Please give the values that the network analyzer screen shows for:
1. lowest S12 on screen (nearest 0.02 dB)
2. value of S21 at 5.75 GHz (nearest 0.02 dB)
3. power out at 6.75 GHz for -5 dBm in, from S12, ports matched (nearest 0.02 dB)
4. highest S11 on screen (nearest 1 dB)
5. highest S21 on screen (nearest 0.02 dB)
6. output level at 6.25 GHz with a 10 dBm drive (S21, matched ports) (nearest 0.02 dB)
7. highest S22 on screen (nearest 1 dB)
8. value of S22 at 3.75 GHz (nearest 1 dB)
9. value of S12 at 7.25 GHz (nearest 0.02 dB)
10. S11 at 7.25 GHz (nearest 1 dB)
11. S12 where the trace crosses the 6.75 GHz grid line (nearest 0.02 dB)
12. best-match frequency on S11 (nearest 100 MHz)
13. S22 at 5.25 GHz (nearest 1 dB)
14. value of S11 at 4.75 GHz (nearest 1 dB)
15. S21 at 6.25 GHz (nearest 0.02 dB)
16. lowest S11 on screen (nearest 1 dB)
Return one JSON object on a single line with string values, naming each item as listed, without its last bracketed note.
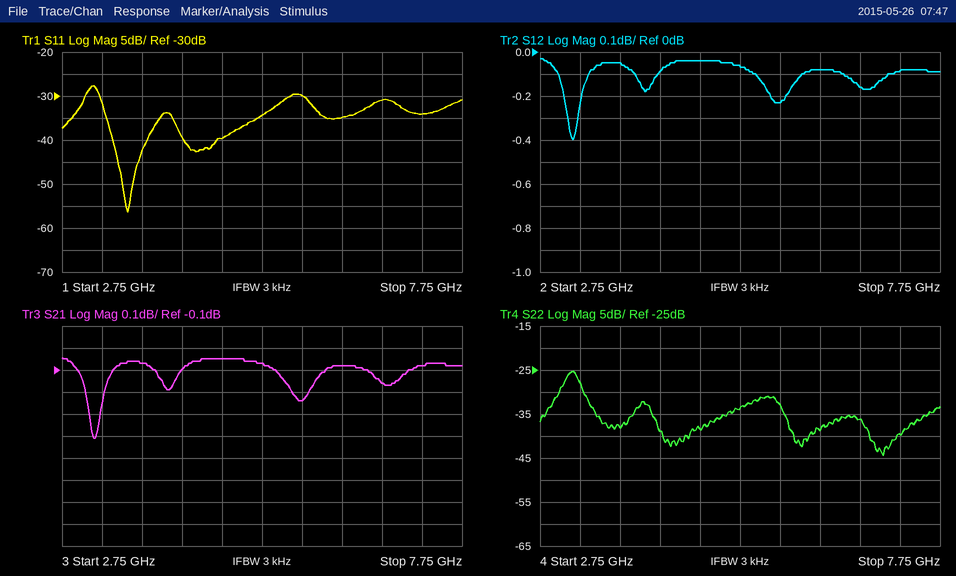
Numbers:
{"lowest S12 on screen": "-0.40 dB", "value of S21 at 5.75 GHz": "-0.24 dB", "power out at 6.75 GHz for -5 dBm in, from S12, ports matched": "-5.16 dBm", "highest S11 on screen": "-28 dB", "highest S21 on screen": "-0.04 dB", "output level at 6.25 GHz with a 10 dBm drive (S21, matched ports)": "9.92 dBm", "highest S22 on screen": "-25 dB", "value of S22 at 3.75 GHz": "-38 dB", "value of S12 at 7.25 GHz": "-0.08 dB", "S11 at 7.25 GHz": "-34 dB", "S12 where the trace crosses the 6.75 GHz grid line": "-0.16 dB", "best-match frequency on S11": "3.6 GHz", "S22 at 5.25 GHz": "-34 dB", "value of S11 at 4.75 GHz": "-40 dB", "S21 at 6.25 GHz": "-0.08 dB", "lowest S11 on screen": "-56 dB"}
